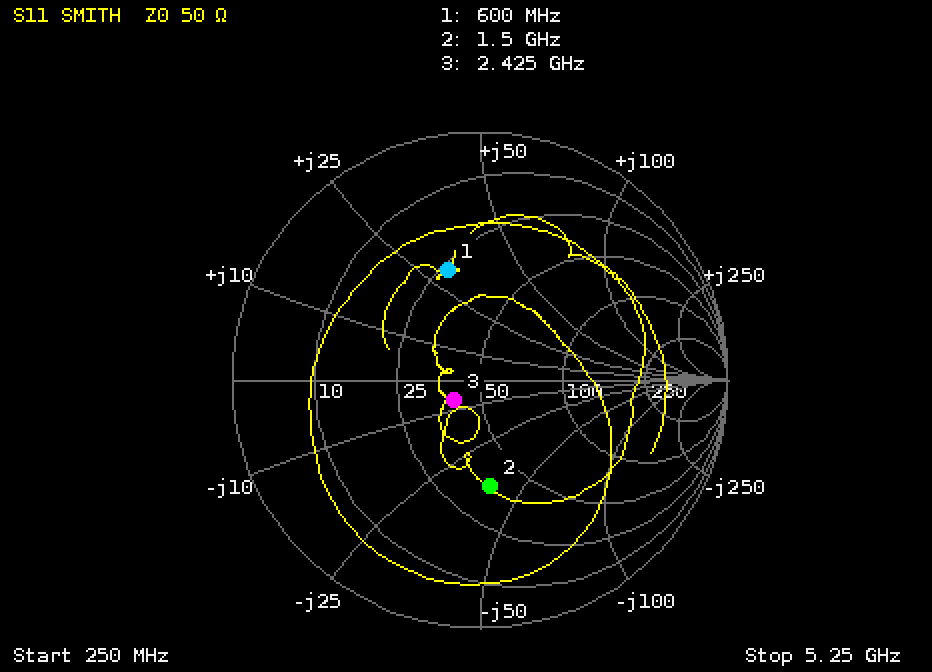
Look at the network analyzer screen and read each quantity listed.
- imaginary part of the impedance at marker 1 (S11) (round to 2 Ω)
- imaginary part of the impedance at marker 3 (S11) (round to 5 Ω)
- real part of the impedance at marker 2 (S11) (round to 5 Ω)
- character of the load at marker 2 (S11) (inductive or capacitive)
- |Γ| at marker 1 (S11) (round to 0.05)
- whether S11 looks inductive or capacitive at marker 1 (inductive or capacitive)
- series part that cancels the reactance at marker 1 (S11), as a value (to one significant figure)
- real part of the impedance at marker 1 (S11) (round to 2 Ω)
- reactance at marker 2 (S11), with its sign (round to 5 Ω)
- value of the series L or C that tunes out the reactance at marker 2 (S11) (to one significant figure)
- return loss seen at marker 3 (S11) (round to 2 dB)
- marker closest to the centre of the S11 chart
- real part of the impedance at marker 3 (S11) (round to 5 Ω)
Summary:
+30 Ω
-5 Ω
35 Ω
capacitive
0.45
inductive
9 pF
26 Ω
-40 Ω
4 nH
18 dB
marker 3
40 Ω
